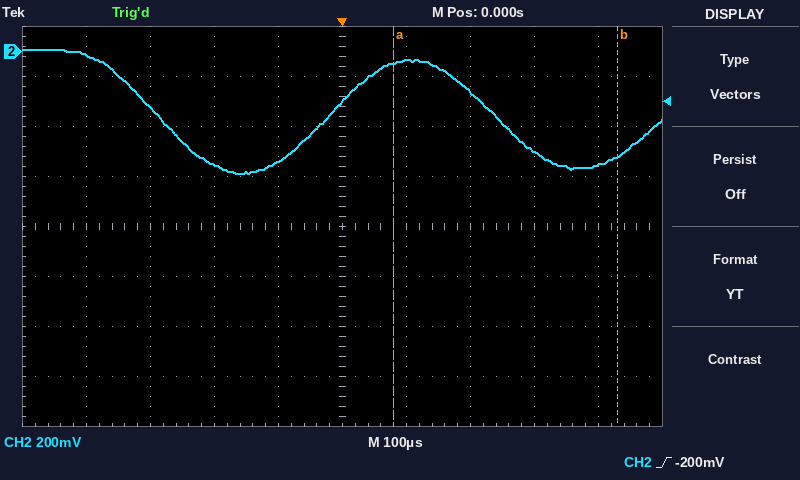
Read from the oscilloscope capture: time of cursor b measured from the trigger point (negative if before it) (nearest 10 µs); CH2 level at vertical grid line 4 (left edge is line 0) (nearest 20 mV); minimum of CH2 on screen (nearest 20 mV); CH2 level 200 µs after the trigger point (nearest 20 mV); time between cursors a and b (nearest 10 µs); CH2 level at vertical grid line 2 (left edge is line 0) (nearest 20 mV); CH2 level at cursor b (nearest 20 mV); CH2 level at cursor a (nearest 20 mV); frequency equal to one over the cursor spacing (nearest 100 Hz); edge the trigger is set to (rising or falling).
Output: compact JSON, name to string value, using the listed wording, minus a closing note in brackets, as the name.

{"time of cursor b measured from the trigger point (negative if before it)": "+430 µs", "CH2 level at vertical grid line 4 (left edge is line 0)": "-440 mV", "minimum of CH2 on screen": "-480 mV", "CH2 level 200 µs after the trigger point": "-160 mV", "time between cursors a and b": "350 µs", "CH2 level at vertical grid line 2 (left edge is line 0)": "-220 mV", "CH2 level at cursor b": "-420 mV", "CH2 level at cursor a": "-40 mV", "frequency equal to one over the cursor spacing": "2.9 kHz", "edge the trigger is set to": "rising"}
